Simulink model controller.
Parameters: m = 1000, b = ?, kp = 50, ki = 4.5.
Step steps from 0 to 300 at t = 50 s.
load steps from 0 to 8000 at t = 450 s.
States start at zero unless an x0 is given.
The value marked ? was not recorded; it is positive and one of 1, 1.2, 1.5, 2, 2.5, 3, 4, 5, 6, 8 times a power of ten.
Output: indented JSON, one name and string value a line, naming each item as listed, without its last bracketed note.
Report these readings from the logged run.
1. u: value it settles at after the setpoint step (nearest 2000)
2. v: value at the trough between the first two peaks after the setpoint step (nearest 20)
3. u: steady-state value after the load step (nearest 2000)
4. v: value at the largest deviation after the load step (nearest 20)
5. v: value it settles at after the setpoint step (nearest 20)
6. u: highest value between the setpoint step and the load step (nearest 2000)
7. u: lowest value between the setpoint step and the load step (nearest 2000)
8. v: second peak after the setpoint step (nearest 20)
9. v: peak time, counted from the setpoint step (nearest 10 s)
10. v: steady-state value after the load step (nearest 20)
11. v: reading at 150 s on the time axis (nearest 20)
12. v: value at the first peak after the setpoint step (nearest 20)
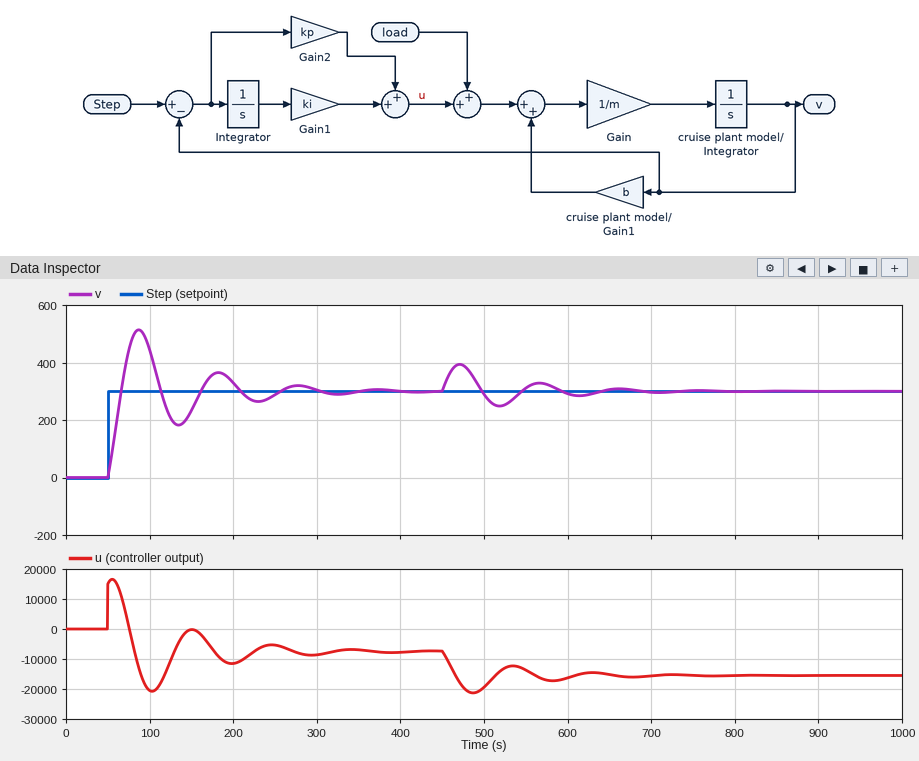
{
  "u: value it settles at after the setpoint step": "-8000",
  "v: value at the trough between the first two peaks after the setpoint step": "180",
  "u: steady-state value after the load step": "-16000",
  "v: value at the largest deviation after the load step": "400",
  "v: value it settles at after the setpoint step": "300",
  "u: highest value between the setpoint step and the load step": "16000",
  "u: lowest value between the setpoint step and the load step": "-20000",
  "v: second peak after the setpoint step": "360",
  "v: peak time, counted from the setpoint step": "40 s",
  "v: steady-state value after the load step": "300",
  "v: reading at 150 s on the time axis": "240",
  "v: value at the first peak after the setpoint step": "520"
}
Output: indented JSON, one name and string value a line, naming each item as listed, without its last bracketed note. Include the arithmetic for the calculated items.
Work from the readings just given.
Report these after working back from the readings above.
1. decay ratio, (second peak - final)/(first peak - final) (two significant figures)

{
  "decay ratio, (second peak - final)/(first peak - final)": "(360 - 300) / (520 - 300) = 0.27"
}
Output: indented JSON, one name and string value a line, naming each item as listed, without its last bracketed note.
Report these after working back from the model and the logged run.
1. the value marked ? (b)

{
  "the value marked ?": "25"
}
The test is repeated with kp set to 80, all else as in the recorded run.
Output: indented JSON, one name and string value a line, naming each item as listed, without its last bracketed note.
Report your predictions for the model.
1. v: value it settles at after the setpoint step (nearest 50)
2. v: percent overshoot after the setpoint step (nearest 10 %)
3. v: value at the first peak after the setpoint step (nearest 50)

{
  "v: value it settles at after the setpoint step": "300",
  "v: percent overshoot after the setpoint step": "50 %",
  "v: value at the first peak after the setpoint step": "450"
}
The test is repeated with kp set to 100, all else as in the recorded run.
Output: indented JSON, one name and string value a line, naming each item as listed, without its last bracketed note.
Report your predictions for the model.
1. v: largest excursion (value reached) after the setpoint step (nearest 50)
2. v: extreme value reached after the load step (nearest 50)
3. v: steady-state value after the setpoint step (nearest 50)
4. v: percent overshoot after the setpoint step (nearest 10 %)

{
  "v: largest excursion (value reached) after the setpoint step": "400",
  "v: extreme value reached after the load step": "350",
  "v: steady-state value after the setpoint step": "300",
  "v: percent overshoot after the setpoint step": "40 %"
}
